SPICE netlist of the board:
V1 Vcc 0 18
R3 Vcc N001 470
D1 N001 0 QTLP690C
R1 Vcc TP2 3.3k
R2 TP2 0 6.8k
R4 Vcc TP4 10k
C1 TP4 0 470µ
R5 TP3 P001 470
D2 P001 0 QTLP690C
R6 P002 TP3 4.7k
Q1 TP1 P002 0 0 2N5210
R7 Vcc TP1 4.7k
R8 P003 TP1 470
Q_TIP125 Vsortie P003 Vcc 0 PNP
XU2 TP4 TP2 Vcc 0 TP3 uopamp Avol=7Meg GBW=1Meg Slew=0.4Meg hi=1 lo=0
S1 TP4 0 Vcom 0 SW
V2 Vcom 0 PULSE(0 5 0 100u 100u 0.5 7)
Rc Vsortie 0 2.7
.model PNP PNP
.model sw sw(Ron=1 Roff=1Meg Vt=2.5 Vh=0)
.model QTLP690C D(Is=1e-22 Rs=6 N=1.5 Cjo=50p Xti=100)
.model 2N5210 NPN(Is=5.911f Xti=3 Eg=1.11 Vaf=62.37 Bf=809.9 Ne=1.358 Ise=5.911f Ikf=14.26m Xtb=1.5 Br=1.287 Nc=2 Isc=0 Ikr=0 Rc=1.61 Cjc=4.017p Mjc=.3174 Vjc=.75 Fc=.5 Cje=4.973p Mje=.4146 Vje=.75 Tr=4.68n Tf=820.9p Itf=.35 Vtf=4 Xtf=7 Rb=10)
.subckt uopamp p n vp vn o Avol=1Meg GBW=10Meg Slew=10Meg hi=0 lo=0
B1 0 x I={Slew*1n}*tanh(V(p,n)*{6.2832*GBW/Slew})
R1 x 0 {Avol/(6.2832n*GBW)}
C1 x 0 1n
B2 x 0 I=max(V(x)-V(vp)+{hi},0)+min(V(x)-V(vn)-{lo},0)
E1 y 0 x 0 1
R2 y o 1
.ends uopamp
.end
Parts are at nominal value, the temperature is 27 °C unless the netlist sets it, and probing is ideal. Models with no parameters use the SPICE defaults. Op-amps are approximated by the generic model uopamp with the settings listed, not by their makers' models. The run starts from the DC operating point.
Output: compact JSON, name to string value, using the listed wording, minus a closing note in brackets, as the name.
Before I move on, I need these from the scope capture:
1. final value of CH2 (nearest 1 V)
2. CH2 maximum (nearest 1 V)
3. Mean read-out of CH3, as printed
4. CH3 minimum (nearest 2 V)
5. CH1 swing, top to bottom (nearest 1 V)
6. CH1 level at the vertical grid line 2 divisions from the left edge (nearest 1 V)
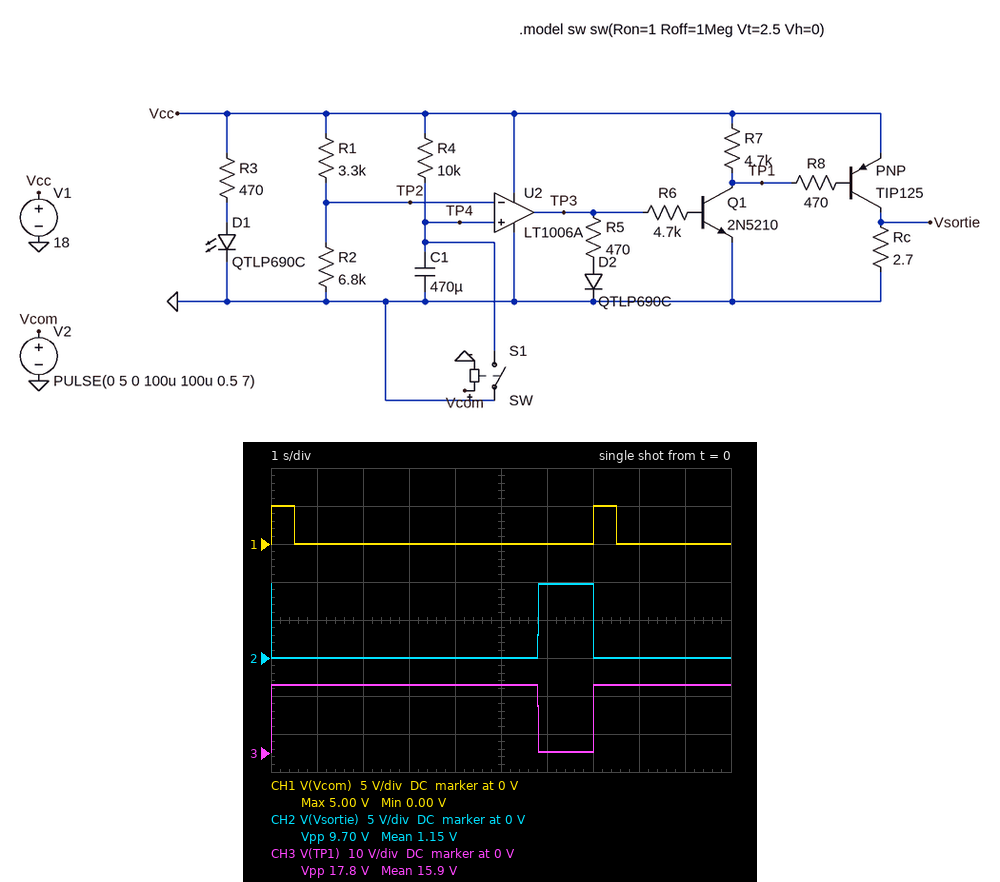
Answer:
{"final value of CH2": "0 V", "CH2 maximum": "10 V", "Mean read-out of CH3, as printed": "15.9 V", "CH3 minimum": "0 V", "CH1 swing, top to bottom": "5 V", "CH1 level at the vertical grid line 2 divisions from the left edge": "0 V"}
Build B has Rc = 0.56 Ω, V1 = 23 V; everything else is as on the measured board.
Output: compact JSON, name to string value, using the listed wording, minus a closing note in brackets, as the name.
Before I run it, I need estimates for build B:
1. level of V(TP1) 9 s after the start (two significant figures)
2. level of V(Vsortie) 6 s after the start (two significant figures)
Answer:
{"level of V(TP1) 9 s after the start": "23 V", "level of V(Vsortie) 6 s after the start": "2.6 V"}
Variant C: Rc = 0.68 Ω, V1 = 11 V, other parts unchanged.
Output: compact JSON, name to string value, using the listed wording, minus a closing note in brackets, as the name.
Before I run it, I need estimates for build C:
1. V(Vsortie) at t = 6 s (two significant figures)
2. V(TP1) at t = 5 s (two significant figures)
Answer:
{"V(Vsortie) at t = 6 s": "1.4 V", "V(TP1) at t = 5 s": "11 V"}
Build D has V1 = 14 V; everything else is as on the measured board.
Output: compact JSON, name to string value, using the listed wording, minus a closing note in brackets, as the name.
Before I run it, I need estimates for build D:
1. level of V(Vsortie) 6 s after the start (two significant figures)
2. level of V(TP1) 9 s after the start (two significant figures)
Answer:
{"level of V(Vsortie) 6 s after the start": "7.4 V", "level of V(TP1) 9 s after the start": "14 V"}
